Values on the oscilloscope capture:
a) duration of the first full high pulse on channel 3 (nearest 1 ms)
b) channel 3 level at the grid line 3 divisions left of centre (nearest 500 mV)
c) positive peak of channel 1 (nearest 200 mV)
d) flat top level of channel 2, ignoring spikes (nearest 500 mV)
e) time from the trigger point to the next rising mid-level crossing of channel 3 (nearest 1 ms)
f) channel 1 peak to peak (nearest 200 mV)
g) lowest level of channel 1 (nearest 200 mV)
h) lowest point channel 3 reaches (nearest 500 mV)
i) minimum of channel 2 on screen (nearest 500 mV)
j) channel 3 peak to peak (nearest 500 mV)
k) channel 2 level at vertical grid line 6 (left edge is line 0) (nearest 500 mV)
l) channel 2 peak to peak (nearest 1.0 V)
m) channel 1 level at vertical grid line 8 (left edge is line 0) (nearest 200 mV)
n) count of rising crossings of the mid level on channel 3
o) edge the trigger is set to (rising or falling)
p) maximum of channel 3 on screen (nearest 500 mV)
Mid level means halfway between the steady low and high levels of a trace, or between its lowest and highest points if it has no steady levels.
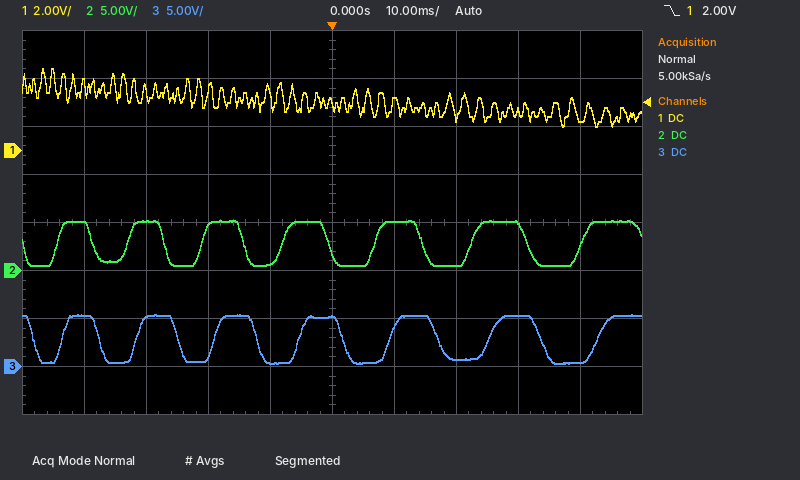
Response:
6 ms
5.0 V
3.4 V
5.0 V
9 ms
2.4 V
1.0 V
500 mV
500 mV
5.0 V
5.0 V
5.0 V
1.6 V
7
falling
5.5 V
